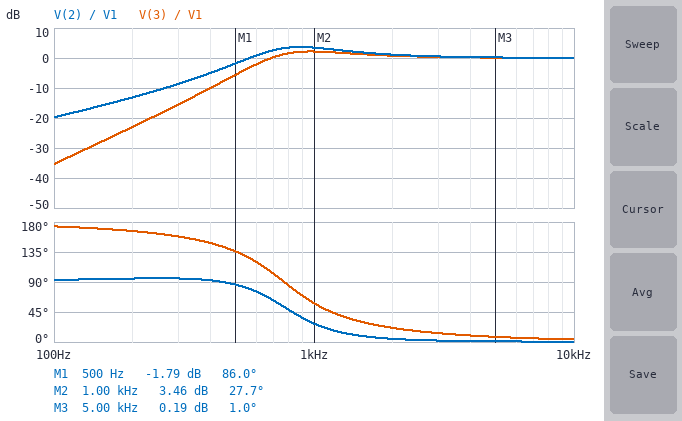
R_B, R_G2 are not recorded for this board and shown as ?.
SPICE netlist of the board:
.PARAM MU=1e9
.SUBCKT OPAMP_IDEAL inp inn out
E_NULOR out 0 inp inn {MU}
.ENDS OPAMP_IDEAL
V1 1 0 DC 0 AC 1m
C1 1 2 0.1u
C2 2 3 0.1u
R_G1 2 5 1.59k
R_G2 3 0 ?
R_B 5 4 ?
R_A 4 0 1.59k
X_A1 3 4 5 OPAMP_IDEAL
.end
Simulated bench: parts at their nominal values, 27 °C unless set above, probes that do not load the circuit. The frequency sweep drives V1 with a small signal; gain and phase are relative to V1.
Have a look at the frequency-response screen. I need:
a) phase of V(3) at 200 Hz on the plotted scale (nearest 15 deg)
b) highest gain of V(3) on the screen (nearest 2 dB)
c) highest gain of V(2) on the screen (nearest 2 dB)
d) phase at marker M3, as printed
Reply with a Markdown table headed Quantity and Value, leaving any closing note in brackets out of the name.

| Quantity | Value |
|---|---|
| phase of V(3) at 200 Hz on the plotted scale | 165 deg |
| highest gain of V(3) on the screen | 2 dB |
| highest gain of V(2) on the screen | 4 dB |
| phase at marker M3, as printed | 1.0 deg |
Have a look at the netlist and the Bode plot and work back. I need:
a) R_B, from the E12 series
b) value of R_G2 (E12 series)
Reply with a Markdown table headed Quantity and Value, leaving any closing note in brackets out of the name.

| Quantity | Value |
|---|---|
| R_B, from the E12 series | 820 Ω |
| value of R_G2 | 2.7 kΩ |
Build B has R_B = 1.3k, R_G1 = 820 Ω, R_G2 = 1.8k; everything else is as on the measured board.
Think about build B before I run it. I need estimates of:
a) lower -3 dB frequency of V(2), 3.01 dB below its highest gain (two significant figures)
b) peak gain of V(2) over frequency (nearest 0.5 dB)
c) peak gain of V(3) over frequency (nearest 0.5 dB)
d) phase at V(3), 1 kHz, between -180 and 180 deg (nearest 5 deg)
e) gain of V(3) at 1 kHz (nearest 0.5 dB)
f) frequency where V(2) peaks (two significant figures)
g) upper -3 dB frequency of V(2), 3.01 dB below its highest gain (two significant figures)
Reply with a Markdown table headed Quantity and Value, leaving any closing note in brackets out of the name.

| Quantity | Value |
|---|---|
| lower -3 dB frequency of V(2), 3.01 dB below its highest gain | 1.2 kHz |
| peak gain of V(2) over frequency | 19.0 dB |
| peak gain of V(3) over frequency | 17.0 dB |
| phase at V(3), 1 kHz, between -180 and 180 deg | 165 deg |
| gain of V(3) at 1 kHz | 2.5 dB |
| frequency where V(2) peaks | 1.3 kHz |
| upper -3 dB frequency of V(2), 3.01 dB below its highest gain | 1.4 kHz |
